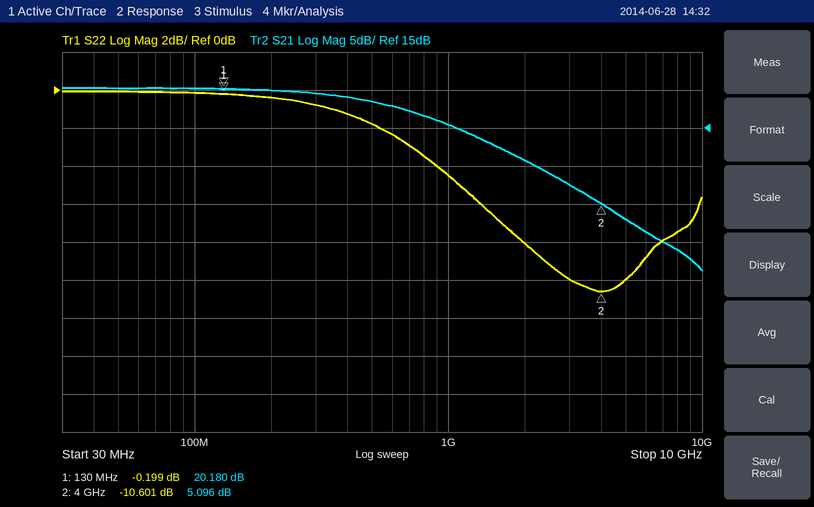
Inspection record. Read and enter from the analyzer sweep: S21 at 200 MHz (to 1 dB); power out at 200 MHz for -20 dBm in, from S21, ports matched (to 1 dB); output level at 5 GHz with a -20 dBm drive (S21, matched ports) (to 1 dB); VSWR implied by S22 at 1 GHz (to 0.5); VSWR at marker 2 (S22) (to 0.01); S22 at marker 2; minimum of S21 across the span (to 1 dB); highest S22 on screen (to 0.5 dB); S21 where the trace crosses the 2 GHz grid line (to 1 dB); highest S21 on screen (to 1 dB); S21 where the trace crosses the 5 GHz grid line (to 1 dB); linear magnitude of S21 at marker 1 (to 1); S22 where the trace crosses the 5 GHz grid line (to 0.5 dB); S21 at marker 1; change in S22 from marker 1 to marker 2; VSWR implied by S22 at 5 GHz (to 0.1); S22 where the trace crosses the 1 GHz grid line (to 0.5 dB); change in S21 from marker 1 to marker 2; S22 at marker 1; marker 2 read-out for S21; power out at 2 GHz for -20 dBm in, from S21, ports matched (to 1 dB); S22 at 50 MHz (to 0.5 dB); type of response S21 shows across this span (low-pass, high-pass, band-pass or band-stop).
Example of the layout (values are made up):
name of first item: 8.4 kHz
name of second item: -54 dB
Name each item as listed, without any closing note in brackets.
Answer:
S21 at 200 MHz: 20 dB
power out at 200 MHz for -20 dBm in, from S21, ports matched: 0 dBm
output level at 5 GHz with a -20 dBm drive (S21, matched ports): -17 dBm
VSWR implied by S22 at 1 GHz: 4.0
VSWR at marker 2 (S22): 1.84
S22 at marker 2: -10.601 dB
minimum of S21 across the span: -4 dB
highest S22 on screen: 0.0 dB
S21 where the trace crosses the 2 GHz grid line: 11 dB
highest S21 on screen: 20 dB
S21 where the trace crosses the 5 GHz grid line: 3 dB
linear magnitude of S21 at marker 1: 10
S22 where the trace crosses the 5 GHz grid line: -10.0 dB
S21 at marker 1: 20.180 dB
change in S22 from marker 1 to marker 2: -10.402 dB
VSWR implied by S22 at 5 GHz: 1.9
S22 where the trace crosses the 1 GHz grid line: -4.5 dB
change in S21 from marker 1 to marker 2: -15.084 dB
S22 at marker 1: -0.199 dB
marker 2 read-out for S21: 5.096 dB
power out at 2 GHz for -20 dBm in, from S21, ports matched: -9 dBm
S22 at 50 MHz: 0.0 dB
type of response S21 shows across this span: low-pass
